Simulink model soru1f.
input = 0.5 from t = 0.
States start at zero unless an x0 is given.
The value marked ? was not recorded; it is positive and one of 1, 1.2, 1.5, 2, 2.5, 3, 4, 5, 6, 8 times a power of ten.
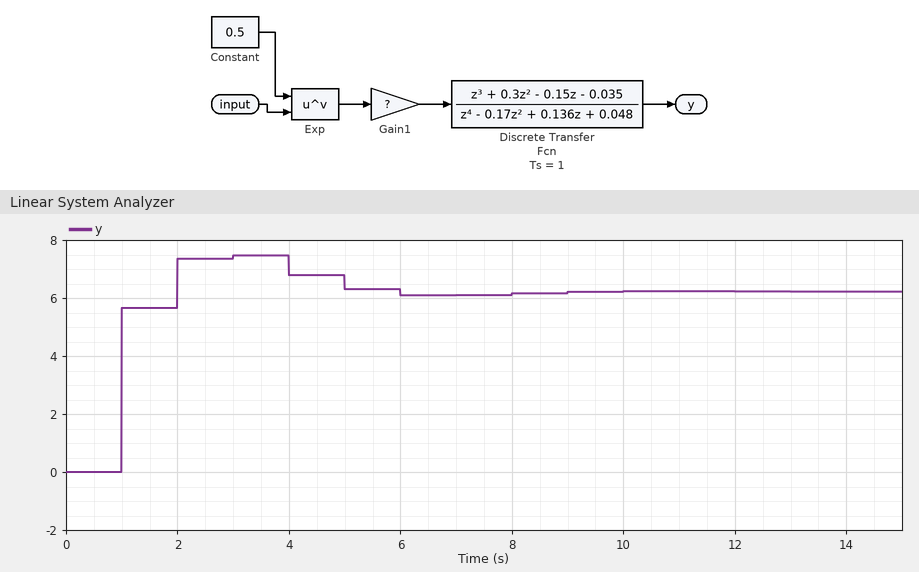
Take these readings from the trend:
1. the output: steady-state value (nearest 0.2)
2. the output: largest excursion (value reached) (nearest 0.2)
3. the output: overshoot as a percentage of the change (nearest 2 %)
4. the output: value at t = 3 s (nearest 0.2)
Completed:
6.2
7.4
20 %
7.4
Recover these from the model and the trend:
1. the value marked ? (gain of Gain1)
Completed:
8
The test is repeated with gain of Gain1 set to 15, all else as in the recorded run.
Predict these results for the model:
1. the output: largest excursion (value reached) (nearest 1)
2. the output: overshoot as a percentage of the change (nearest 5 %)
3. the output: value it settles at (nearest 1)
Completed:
14
20 %
12
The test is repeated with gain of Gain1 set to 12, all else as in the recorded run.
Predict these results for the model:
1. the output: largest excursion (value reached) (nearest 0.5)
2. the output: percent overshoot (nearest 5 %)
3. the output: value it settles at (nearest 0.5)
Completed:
11.0
20 %
9.5
